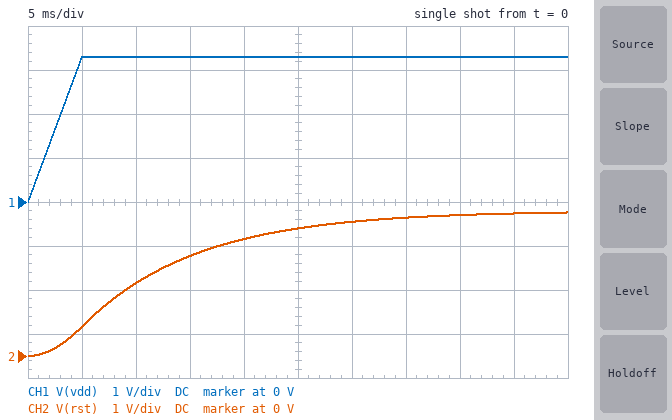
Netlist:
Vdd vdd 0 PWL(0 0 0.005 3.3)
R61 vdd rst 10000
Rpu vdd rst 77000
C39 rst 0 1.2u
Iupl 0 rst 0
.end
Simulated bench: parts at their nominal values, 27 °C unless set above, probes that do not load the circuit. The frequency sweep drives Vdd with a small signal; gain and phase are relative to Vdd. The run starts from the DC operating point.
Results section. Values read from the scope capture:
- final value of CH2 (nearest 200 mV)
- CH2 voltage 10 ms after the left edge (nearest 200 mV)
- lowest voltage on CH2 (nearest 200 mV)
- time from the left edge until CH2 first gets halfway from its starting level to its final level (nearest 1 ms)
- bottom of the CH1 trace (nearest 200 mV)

3.2 V
1.6 V
0 V
10 ms
0 V
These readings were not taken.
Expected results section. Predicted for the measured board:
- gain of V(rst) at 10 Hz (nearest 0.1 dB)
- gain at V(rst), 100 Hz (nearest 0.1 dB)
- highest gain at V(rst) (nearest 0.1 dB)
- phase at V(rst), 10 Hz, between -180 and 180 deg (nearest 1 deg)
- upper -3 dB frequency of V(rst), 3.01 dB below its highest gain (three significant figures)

-1.6 dB
-16.6 dB
0 dB
-34 deg
15.0 Hz
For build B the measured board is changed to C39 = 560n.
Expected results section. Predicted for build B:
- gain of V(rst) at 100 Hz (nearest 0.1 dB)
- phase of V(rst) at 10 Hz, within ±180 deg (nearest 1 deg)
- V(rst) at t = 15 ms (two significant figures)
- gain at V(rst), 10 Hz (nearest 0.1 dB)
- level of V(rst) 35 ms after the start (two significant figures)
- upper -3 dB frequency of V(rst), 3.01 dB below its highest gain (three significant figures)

-10.3 dB
-17 deg
3.0 V
-0.4 dB
3.3 V
32.1 Hz
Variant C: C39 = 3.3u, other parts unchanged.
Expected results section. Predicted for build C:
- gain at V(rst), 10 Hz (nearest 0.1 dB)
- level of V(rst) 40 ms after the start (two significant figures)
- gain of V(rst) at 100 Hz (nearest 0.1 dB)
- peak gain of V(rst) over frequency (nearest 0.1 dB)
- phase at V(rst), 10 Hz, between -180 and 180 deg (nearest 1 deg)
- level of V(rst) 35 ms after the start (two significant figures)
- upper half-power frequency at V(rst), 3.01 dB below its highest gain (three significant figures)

-6.4 dB
2.4 V
-25.3 dB
0 dB
-61 deg
2.2 V
5.45 Hz
